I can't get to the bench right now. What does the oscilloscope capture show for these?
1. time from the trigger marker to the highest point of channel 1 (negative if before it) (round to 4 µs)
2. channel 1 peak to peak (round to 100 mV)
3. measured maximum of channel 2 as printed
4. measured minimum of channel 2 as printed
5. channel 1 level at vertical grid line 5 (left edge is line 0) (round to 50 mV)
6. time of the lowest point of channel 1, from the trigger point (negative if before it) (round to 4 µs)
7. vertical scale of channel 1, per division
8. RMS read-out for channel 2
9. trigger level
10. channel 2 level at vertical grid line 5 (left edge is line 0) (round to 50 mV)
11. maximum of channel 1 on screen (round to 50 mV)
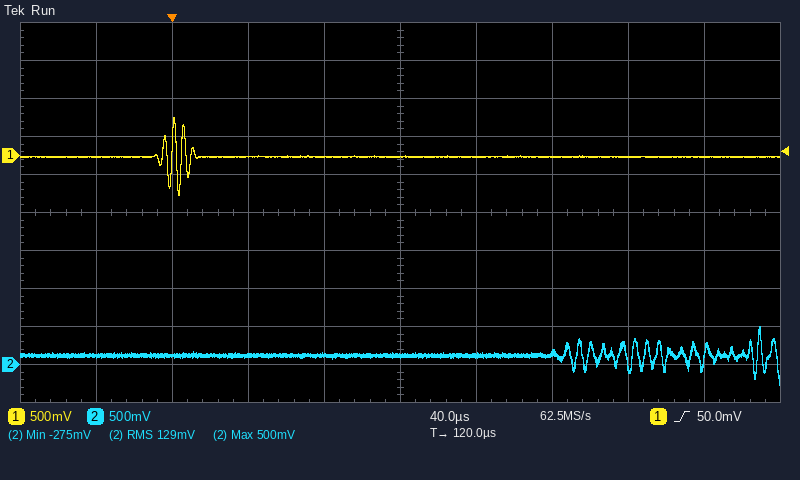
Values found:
0 µs
1.00 V
500 mV
-275 mV
0 mV
+4 µs
500 mV
129 mV
50.0 mV
100 mV
500 mV
